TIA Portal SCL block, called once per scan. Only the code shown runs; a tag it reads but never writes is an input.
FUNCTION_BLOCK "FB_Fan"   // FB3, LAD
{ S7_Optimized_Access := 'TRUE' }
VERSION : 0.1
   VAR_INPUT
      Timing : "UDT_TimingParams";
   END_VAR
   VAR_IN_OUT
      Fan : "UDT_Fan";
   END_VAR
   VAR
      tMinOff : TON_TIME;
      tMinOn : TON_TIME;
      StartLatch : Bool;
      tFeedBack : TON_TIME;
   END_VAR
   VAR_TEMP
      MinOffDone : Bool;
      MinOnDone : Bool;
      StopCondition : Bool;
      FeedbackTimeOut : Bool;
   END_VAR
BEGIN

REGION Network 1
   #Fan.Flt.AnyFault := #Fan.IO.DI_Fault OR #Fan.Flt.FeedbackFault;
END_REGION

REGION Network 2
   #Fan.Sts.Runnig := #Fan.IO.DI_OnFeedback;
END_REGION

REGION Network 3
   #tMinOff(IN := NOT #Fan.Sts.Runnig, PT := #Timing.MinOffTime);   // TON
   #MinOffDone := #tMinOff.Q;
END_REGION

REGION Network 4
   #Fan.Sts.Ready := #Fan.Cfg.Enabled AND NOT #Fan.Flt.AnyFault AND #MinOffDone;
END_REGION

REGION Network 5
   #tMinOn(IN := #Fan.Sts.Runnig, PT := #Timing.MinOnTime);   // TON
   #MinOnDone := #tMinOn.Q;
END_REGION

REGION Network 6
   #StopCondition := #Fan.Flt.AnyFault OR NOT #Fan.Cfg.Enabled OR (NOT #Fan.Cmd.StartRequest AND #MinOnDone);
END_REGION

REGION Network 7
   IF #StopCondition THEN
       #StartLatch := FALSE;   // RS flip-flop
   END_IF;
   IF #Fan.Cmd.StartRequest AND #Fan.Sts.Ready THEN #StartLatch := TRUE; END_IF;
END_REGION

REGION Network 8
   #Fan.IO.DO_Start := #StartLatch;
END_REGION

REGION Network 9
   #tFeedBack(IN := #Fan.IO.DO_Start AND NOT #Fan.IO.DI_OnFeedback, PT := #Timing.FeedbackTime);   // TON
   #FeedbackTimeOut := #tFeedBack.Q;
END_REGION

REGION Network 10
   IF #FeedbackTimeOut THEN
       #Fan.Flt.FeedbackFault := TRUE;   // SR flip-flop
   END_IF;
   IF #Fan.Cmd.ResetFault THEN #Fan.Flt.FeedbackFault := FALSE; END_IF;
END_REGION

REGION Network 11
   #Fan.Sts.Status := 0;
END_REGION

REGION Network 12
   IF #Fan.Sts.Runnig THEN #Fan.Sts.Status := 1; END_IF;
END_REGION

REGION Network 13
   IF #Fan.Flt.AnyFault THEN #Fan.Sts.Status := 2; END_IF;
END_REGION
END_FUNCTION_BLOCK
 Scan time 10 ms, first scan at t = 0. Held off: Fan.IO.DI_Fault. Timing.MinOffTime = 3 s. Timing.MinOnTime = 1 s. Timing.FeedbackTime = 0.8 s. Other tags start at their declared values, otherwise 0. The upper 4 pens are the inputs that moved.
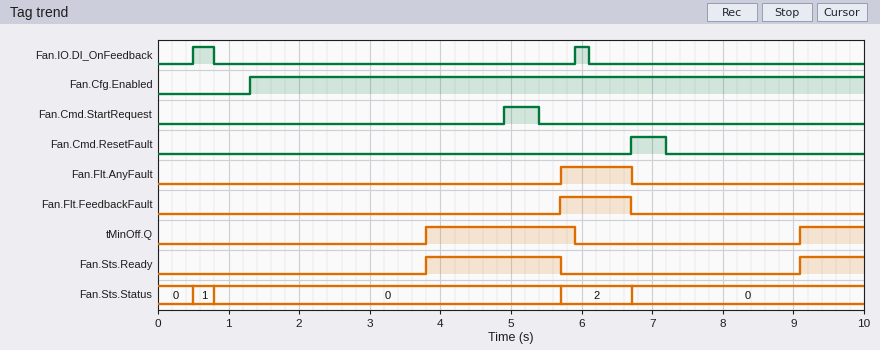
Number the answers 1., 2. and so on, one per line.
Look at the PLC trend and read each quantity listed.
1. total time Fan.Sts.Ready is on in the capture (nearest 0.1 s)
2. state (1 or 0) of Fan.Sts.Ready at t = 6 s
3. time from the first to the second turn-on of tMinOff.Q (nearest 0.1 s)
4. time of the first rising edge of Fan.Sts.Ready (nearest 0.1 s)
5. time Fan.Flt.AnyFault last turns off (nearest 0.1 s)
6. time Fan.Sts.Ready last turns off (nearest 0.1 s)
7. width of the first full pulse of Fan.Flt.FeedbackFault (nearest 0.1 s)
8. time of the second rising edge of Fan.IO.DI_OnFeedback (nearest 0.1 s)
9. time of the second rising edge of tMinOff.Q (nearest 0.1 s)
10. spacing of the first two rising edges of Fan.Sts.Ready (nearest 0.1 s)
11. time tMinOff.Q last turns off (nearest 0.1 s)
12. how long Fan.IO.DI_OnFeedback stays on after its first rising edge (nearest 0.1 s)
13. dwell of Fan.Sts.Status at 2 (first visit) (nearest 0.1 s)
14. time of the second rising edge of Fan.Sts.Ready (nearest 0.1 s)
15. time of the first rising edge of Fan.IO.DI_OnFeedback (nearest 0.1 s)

1. 2.8 s
2. 0
3. 5.3 s
4. 3.8 s
5. 6.7 s
6. 5.7 s
7. 1.0 s
8. 5.9 s
9. 9.1 s
10. 5.3 s
11. 5.9 s
12. 0.3 s
13. 1.0 s
14. 9.1 s
15. 0.5 s
